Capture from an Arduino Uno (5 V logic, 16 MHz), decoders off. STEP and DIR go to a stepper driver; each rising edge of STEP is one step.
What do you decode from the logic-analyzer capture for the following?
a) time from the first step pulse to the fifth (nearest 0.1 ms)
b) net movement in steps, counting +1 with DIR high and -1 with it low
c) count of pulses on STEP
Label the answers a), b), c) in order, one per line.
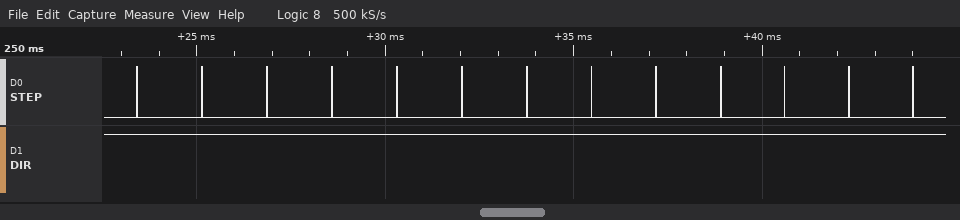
a) 6.9 ms
b) +13
c) 13
